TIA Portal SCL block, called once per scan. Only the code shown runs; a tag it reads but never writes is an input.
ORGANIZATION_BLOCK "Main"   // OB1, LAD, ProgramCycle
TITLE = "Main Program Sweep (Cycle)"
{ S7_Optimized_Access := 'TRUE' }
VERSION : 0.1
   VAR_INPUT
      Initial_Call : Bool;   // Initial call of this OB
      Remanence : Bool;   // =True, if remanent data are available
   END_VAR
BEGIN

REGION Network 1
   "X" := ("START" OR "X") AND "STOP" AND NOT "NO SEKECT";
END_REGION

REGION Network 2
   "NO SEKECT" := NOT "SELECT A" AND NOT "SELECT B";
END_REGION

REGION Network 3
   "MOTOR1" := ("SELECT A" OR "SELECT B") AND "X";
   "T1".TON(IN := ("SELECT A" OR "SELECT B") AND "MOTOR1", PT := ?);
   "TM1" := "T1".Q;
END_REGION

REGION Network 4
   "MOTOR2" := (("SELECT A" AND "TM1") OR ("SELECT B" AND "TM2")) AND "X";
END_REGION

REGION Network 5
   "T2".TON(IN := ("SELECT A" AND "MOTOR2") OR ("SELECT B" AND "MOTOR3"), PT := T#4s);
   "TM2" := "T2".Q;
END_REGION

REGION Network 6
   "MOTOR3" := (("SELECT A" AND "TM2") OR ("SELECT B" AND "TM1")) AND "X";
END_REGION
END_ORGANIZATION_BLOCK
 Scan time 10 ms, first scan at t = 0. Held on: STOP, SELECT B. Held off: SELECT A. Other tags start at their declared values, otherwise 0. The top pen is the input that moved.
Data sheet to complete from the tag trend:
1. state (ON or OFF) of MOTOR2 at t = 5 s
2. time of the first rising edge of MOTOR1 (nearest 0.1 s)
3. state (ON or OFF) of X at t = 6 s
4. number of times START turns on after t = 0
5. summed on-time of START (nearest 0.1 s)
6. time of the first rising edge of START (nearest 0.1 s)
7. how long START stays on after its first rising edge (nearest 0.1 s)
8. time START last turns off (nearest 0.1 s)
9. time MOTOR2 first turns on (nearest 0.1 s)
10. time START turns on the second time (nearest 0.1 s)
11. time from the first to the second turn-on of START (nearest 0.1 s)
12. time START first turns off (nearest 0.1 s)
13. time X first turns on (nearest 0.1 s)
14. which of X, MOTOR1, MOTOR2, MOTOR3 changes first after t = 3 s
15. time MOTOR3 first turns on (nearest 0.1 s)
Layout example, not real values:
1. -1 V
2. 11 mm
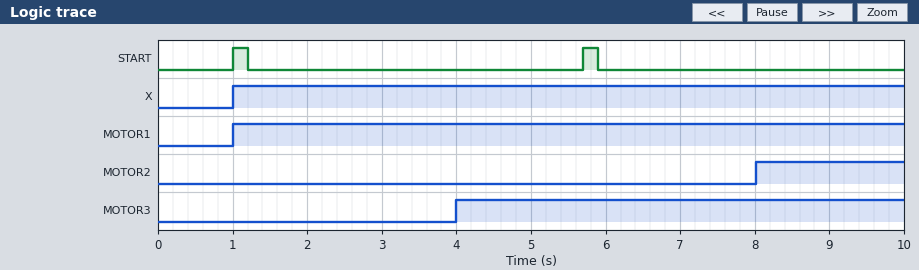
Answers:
1. OFF
2. 1.0 s
3. ON
4. 2
5. 0.4 s
6. 1.0 s
7. 0.2 s
8. 5.9 s
9. 8.0 s
10. 5.7 s
11. 4.7 s
12. 1.2 s
13. 1.0 s
14. MOTOR3
15. 4.0 s
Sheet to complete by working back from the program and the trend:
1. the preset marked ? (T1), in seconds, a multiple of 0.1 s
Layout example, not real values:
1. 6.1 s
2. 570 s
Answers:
1. 3.0 s
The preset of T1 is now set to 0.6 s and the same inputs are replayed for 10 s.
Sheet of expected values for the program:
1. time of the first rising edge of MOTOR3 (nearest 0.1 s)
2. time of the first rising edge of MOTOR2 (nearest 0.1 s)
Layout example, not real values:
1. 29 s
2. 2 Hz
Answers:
1. 1.6 s
2. 5.6 s
